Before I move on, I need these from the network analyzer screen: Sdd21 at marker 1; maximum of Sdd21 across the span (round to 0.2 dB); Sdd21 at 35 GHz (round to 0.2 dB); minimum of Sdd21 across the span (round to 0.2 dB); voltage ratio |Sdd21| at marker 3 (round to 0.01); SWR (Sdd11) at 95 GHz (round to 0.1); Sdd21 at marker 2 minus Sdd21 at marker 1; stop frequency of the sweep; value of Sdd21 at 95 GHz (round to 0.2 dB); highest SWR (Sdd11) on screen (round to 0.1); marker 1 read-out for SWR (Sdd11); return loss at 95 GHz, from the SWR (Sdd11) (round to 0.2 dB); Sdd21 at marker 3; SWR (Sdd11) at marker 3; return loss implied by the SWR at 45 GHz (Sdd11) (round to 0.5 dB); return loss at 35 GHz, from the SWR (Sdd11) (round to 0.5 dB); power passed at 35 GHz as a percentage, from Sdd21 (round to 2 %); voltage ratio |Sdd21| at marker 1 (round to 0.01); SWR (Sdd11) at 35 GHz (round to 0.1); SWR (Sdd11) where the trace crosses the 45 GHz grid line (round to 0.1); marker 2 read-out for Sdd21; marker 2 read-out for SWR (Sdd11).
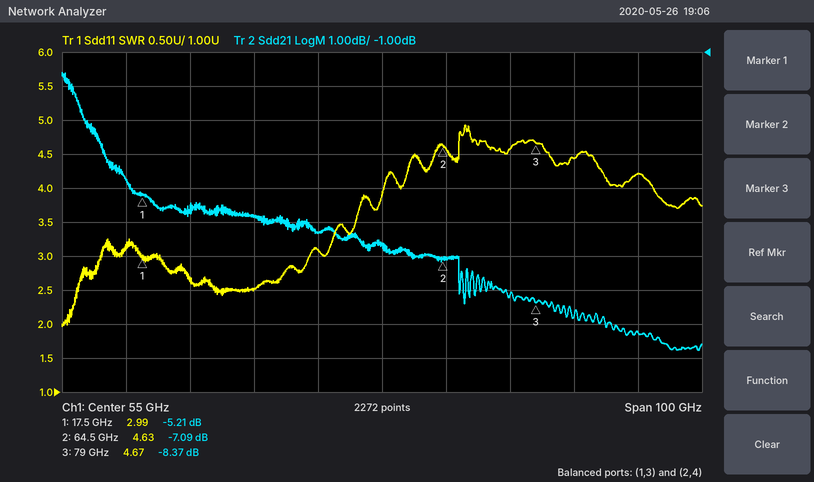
-5.21 dB
-1.6 dB
-5.8 dB
-9.8 dB
0.38
4.2
-1.88 dB
105 GHz
-9.2 dB
4.9
2.99
4.2 dB
-8.37 dB
4.67
6.0 dB
7.5 dB
26 %
0.55
2.5
3.1
-7.09 dB
4.63
